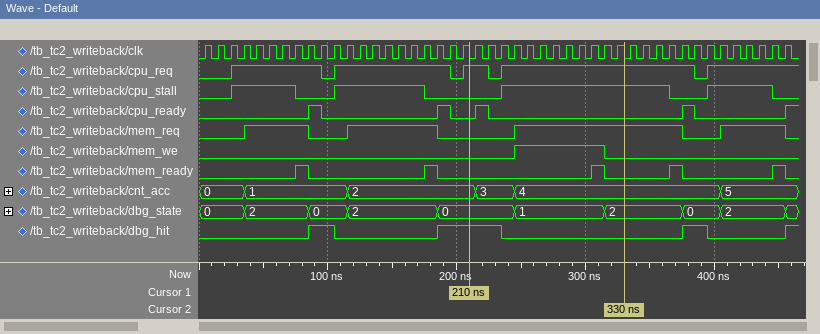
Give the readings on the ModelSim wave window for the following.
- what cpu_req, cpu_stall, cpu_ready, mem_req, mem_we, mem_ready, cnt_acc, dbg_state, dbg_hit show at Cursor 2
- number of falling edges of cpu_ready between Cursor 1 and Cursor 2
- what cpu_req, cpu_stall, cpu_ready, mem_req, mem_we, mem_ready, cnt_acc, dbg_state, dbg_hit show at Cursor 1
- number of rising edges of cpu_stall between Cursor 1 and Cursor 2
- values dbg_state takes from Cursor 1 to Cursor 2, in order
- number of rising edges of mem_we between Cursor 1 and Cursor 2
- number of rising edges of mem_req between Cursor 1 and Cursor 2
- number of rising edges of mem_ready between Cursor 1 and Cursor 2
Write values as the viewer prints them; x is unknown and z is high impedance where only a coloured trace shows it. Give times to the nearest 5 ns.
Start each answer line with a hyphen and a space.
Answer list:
- cpu_req=1, cpu_stall=1, cpu_ready=0, mem_req=1, mem_we=0, mem_ready=0, cnt_acc=4, dbg_state=2, dbg_hit=0
- 1
- cpu_req=1, cpu_stall=0, cpu_ready=0, mem_req=0, mem_we=0, mem_ready=0, cnt_acc=2, dbg_state=0, dbg_hit=1
- 1
- 0, 1, 2
- 1
- 1
- 1
